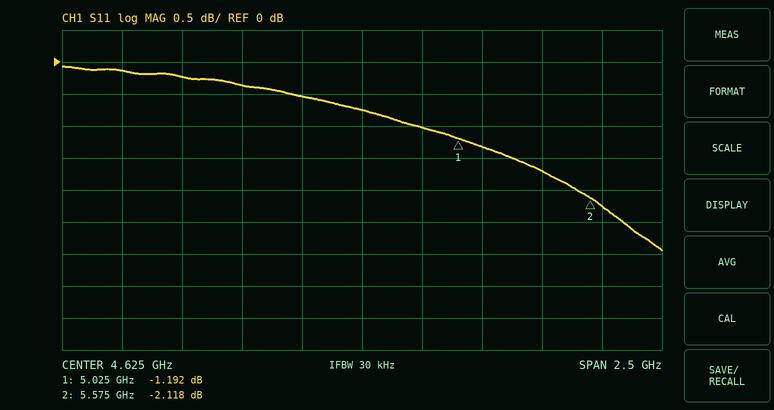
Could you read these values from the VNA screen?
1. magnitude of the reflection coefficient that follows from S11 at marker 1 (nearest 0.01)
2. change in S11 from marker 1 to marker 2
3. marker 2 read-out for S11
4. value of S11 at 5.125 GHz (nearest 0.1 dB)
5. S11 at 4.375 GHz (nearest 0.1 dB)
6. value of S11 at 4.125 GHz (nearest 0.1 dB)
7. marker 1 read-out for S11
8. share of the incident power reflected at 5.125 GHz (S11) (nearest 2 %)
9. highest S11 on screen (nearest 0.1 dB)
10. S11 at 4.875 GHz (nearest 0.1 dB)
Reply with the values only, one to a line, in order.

0.87
-0.926 dB
-2.118 dB
-1.3 dB
-0.5 dB
-0.4 dB
-1.192 dB
74 %
-0.1 dB
-1.0 dB
